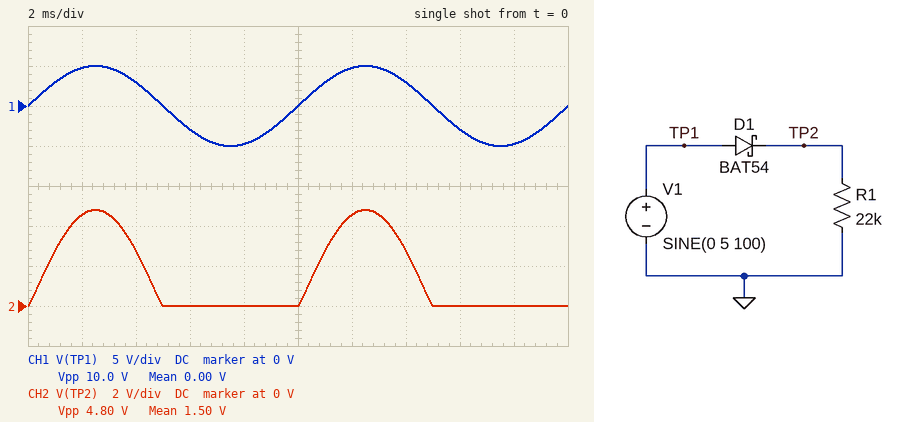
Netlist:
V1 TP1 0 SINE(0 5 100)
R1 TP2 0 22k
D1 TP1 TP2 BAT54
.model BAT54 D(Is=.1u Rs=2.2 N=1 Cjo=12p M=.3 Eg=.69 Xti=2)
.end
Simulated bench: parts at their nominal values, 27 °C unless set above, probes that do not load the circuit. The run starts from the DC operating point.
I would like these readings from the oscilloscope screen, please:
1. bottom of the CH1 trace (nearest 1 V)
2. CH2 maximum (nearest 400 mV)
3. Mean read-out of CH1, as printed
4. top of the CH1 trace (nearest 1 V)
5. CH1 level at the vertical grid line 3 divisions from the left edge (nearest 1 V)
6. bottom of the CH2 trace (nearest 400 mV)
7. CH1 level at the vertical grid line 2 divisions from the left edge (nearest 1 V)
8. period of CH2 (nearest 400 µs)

-5 V
4.8 V
0.00 V
5 V
-3 V
0 V
3 V
10.0 ms
